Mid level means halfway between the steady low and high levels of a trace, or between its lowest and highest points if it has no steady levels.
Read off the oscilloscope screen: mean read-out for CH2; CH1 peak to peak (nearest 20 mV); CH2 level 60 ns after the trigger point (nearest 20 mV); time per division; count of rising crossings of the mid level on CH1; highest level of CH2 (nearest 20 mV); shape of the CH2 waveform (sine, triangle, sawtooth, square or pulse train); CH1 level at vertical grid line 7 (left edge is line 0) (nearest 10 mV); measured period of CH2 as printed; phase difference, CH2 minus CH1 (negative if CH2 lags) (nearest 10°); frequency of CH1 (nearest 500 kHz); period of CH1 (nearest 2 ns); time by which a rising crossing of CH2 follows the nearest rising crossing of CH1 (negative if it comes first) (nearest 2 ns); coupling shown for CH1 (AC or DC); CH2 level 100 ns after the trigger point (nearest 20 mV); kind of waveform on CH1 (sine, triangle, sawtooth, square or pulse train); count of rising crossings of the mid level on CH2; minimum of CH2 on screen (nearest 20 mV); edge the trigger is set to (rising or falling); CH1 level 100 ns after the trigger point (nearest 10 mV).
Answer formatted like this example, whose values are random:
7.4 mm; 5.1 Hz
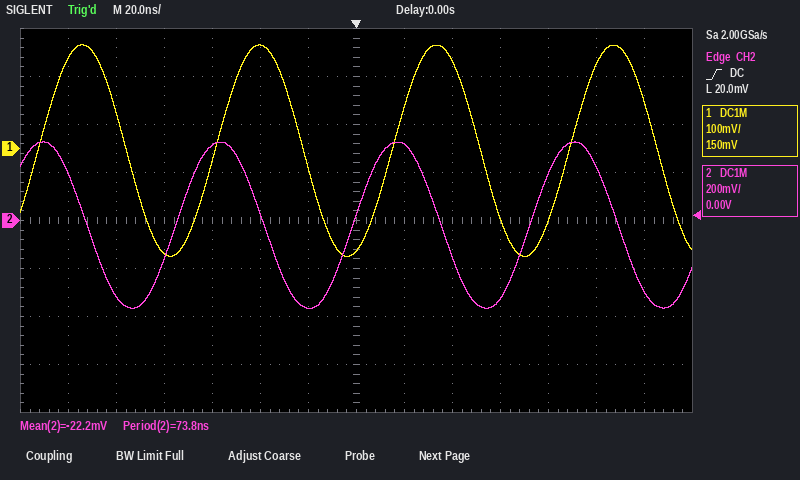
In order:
-22.2 mV; 440 mV; -320 mV; 20 ns; 4; 320 mV; sine; -210 mV; 73.8 ns; +80°; 13.5 MHz; 74 ns; -16 ns; DC; 220 mV; sine; 3; -360 mV; rising; 170 mV
